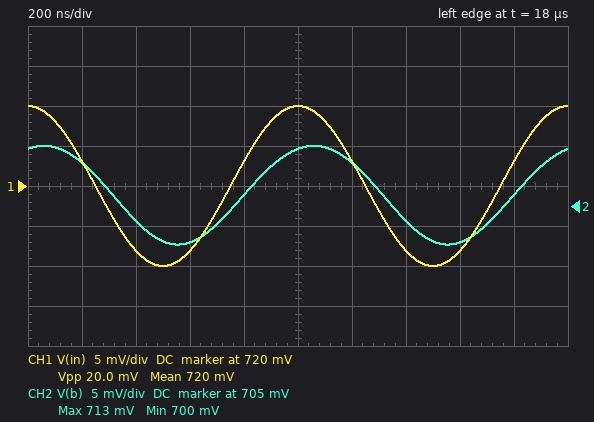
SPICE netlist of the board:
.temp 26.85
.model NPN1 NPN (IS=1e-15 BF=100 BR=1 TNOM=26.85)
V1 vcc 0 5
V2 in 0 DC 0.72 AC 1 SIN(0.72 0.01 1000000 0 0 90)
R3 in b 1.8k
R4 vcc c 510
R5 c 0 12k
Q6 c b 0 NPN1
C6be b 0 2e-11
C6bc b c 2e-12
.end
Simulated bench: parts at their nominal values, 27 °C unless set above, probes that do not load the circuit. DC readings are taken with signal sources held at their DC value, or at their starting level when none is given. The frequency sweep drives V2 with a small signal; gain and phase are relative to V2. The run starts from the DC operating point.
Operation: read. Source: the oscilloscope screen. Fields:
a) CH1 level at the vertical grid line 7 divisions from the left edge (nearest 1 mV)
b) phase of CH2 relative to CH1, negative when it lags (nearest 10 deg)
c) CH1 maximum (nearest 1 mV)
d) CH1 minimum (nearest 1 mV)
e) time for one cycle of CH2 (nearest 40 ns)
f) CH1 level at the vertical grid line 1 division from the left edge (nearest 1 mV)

712 mV
-20 deg
730 mV
710 mV
1.00 µs
723 mV
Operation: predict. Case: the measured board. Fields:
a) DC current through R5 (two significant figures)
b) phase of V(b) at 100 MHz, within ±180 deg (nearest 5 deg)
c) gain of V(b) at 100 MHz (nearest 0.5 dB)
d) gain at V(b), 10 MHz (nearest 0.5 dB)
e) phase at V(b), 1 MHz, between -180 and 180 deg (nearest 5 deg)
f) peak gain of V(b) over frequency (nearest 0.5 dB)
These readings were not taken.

370 µA
-70 deg
-34.0 dB
-15.5 dB
-20 deg
-3.5 dB
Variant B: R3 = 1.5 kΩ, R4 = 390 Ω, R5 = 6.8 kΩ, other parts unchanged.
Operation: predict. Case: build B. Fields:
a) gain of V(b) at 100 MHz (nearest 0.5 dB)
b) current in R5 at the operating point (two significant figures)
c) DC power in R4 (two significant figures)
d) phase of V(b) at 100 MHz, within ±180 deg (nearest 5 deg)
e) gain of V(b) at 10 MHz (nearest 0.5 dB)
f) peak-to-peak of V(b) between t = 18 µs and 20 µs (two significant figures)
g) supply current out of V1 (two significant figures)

-32.0 dB
650 µA
810 µW
-75 deg
-13.0 dB
13 mV
1.4 mA
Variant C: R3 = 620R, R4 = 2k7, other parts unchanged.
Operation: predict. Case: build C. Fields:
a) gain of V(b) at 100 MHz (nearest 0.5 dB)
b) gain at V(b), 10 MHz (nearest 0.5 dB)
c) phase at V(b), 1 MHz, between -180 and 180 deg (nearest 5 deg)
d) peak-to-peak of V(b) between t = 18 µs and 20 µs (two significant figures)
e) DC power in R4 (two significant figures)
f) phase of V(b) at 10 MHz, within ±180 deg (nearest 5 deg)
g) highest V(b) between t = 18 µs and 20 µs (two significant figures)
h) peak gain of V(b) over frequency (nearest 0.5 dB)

-28.5 dB
-17.5 dB
-30 deg
14 mV
3.5 mW
-65 deg
720 mV
-2.0 dB
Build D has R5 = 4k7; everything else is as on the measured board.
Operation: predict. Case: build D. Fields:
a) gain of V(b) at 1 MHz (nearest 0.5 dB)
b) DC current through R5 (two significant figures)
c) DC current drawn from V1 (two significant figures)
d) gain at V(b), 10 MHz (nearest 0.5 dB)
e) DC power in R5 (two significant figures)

-4.0 dB
890 µA
1.6 mA
-15.0 dB
3.7 mW
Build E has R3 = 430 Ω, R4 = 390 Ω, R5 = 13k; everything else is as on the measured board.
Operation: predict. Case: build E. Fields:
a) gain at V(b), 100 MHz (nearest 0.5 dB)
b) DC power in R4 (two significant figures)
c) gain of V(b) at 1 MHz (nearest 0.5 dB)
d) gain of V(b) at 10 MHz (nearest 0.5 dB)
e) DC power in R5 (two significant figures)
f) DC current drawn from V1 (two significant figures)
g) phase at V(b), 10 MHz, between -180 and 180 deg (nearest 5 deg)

-22.5 dB
750 µW
-1.5 dB
-5.5 dB
1.5 mW
1.4 mA
-50 deg
